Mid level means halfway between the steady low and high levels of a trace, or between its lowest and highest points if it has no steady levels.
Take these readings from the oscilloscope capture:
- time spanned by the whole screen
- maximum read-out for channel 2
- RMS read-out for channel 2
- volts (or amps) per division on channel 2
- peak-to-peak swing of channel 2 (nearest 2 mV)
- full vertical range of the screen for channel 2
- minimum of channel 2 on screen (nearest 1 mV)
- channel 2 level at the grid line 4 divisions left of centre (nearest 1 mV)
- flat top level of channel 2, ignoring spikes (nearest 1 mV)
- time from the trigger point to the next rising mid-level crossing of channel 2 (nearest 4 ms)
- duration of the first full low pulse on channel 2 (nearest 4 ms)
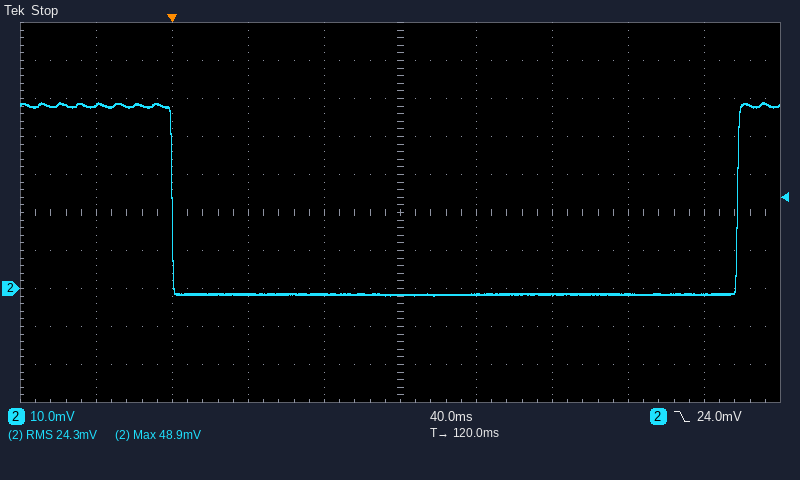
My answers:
400 ms
48.9 mV
24.3 mV
10 mV
50 mV
100 mV
-2 mV
48 mV
48 mV
296 ms
296 ms
